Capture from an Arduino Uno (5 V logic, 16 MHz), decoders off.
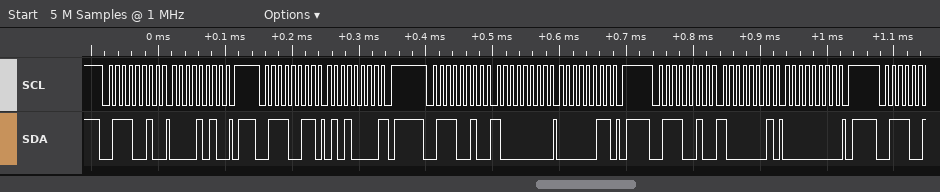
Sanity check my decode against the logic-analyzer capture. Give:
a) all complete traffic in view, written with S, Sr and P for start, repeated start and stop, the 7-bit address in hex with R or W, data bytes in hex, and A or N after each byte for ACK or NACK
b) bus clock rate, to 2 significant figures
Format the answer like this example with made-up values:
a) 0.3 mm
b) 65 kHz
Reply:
a) S 39W A 0A A P S 39R A 50 N P S 39W A 80 A 03 A P S 39W A 81 A 00 A P
b) 100 kHz
